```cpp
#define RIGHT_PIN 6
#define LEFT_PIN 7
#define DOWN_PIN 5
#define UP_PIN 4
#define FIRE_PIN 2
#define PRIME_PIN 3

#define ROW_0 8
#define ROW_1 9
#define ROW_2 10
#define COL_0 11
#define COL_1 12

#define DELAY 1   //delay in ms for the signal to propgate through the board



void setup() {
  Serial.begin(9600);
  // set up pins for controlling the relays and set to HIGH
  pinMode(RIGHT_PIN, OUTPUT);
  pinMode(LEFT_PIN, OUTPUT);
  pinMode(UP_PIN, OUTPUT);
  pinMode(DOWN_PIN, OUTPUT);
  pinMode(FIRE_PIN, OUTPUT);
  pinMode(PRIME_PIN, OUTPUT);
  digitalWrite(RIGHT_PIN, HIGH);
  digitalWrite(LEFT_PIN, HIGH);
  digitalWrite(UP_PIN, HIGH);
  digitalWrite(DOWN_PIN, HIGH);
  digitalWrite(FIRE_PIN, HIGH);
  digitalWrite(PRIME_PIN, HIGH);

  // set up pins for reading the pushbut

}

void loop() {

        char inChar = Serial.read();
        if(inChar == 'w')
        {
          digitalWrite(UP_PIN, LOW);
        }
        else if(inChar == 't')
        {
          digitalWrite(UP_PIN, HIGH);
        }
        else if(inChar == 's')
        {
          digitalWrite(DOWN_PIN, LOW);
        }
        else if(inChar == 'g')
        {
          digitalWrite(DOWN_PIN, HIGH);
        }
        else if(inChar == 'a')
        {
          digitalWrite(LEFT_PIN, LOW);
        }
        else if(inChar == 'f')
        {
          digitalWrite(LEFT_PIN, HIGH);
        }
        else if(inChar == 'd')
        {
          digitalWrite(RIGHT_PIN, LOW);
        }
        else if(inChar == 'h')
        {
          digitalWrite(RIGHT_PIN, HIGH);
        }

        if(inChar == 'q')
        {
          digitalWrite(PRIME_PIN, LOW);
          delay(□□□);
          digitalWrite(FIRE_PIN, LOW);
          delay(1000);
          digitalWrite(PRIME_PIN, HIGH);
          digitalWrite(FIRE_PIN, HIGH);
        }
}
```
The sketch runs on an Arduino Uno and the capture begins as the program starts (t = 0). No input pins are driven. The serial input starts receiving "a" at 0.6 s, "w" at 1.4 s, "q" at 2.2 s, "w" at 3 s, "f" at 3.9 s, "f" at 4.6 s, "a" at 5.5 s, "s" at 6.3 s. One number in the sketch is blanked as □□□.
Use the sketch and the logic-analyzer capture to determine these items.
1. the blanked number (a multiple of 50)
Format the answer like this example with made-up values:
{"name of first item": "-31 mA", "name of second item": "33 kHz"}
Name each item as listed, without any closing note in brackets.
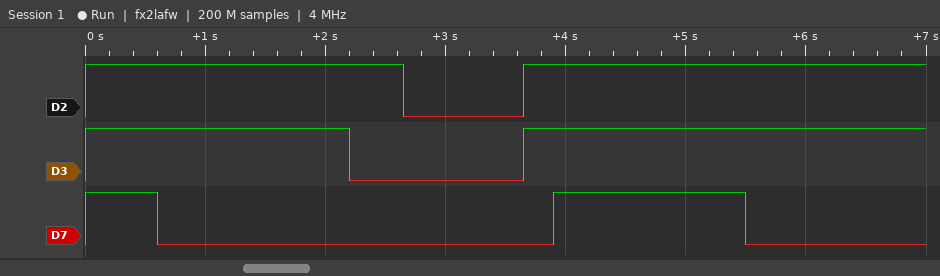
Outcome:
{"the blanked number": "450"}
